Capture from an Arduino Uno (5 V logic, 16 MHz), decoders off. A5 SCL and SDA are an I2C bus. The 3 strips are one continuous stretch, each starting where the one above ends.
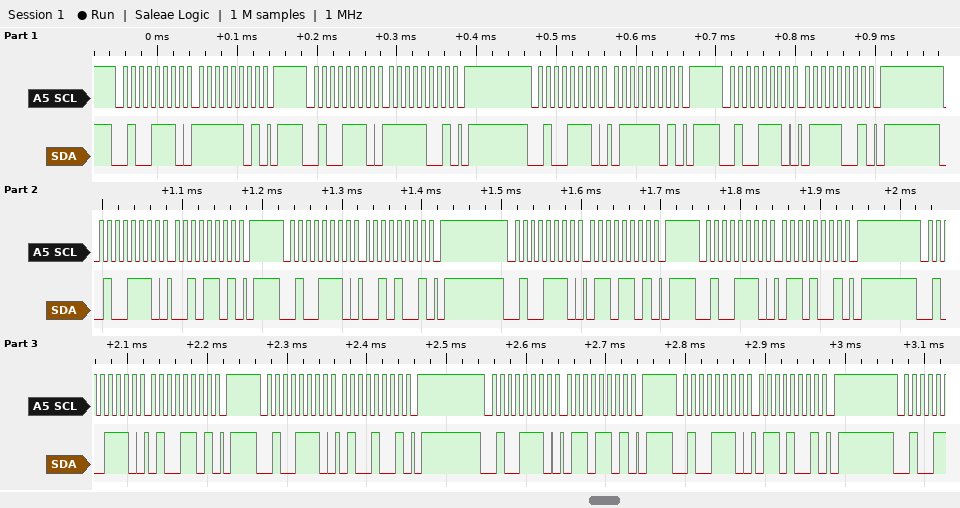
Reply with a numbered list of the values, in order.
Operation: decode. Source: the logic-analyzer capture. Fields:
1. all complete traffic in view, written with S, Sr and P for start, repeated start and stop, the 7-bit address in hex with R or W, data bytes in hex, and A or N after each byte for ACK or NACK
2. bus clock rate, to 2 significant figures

1. S 27W A FD A P S 27W A F9 A P S 27W A 7D A P S 27W A 79 A P S 27W A 2D A P S 27W A 29 A P S 27W A 6D A P S 27W A 69 A P S 27W A 4D A P S 27W A 49 A P S 27W A 6D A P S 27W A 69 A P
2. 100 kHz
